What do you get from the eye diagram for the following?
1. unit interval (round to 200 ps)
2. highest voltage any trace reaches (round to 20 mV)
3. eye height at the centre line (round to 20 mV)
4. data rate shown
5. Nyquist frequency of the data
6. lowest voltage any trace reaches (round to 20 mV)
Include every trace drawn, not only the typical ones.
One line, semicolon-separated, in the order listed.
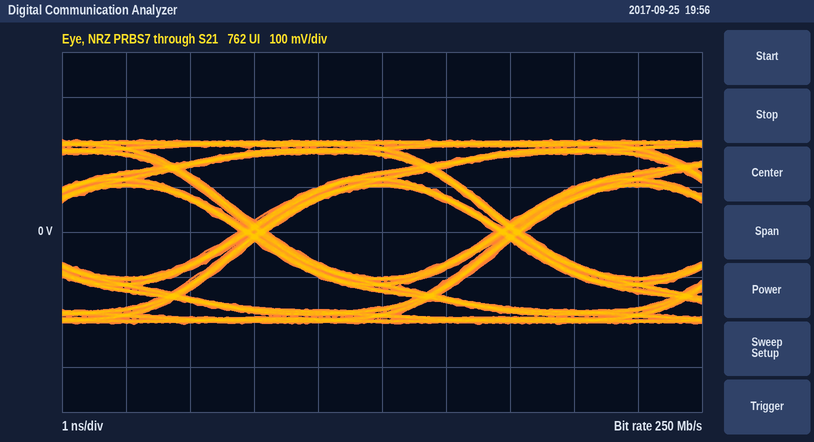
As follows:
4.0 ns; 200 mV; 200 mV; 250 Mb/s; 125 MHz; -200 mV
